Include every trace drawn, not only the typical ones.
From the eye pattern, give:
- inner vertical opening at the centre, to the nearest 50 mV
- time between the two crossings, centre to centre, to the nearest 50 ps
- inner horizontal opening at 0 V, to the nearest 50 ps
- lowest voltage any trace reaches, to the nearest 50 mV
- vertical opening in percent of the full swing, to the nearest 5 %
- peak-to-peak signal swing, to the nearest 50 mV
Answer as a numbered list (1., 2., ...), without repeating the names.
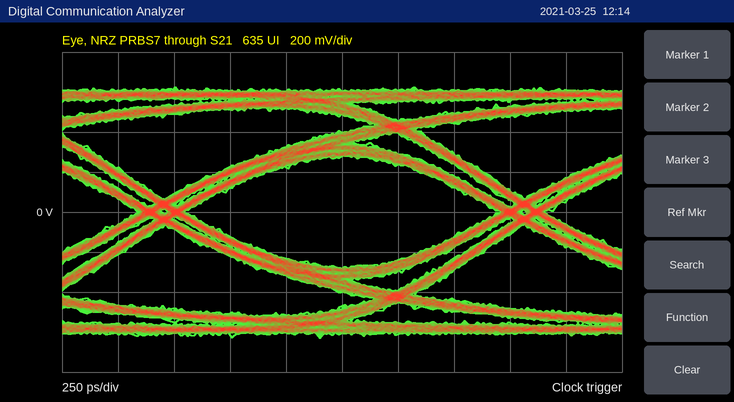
1. 550 mV
2. 1.60 ns
3. 1.40 ns
4. -650 mV
5. 45 %
6. 1.25 V
